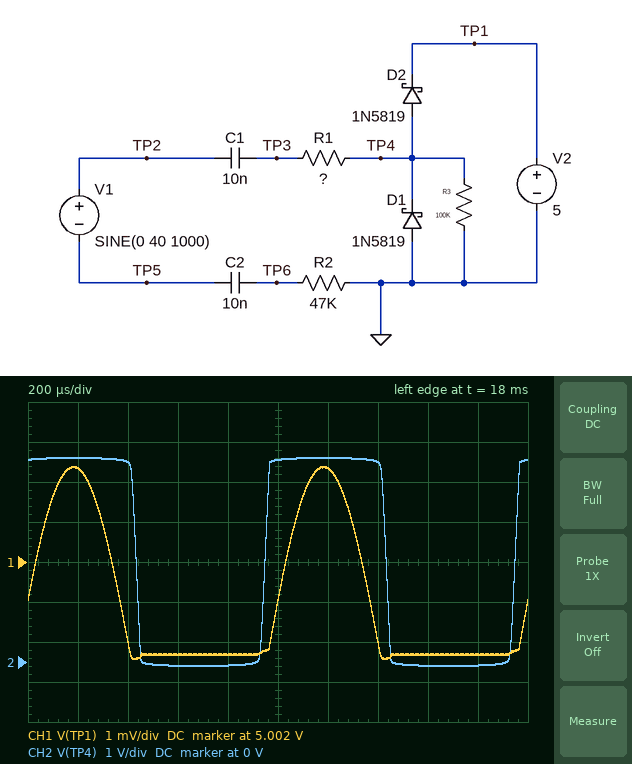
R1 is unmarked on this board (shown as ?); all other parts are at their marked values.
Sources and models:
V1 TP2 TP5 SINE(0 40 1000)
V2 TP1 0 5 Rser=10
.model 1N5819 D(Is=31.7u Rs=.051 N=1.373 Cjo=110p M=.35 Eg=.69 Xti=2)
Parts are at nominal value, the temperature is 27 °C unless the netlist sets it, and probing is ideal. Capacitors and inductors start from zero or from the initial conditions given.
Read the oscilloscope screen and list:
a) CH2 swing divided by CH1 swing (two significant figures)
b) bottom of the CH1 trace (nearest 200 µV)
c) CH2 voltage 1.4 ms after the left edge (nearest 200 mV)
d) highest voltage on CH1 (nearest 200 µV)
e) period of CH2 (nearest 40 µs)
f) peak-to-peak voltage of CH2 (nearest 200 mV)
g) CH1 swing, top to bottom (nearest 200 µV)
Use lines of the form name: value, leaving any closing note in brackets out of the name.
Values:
CH2 swing divided by CH1 swing: 1100
bottom of the CH1 trace: 4.9996 V
CH2 voltage 1.4 ms after the left edge: 5.0 V
highest voltage on CH1: 5.0044 V
period of CH2: 1.00 ms
peak-to-peak voltage of CH2: 5.2 V
CH1 swing, top to bottom: 4.8 mV
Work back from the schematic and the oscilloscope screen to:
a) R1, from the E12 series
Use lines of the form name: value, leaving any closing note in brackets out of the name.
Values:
R1, from the E12 series: 18 kΩ
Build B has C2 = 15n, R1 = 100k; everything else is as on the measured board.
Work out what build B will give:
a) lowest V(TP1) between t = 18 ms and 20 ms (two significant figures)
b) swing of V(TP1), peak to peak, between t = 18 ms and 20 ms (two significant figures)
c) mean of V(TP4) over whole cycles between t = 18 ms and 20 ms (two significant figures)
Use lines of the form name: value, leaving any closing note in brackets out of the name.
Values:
lowest V(TP1) between t = 18 ms and 20 ms: 5.0 V
swing of V(TP1), peak to peak, between t = 18 ms and 20 ms: 2.1 mV
mean of V(TP4) over whole cycles between t = 18 ms and 20 ms: 2.3 V
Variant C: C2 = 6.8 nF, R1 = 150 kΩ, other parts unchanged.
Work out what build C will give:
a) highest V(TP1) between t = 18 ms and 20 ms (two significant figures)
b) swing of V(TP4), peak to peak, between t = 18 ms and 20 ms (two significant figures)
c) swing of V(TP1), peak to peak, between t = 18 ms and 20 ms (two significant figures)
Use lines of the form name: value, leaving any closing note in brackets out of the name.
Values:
highest V(TP1) between t = 18 ms and 20 ms: 5.0 V
swing of V(TP4), peak to peak, between t = 18 ms and 20 ms: 5.1 V
swing of V(TP1), peak to peak, between t = 18 ms and 20 ms: 1.4 mV
